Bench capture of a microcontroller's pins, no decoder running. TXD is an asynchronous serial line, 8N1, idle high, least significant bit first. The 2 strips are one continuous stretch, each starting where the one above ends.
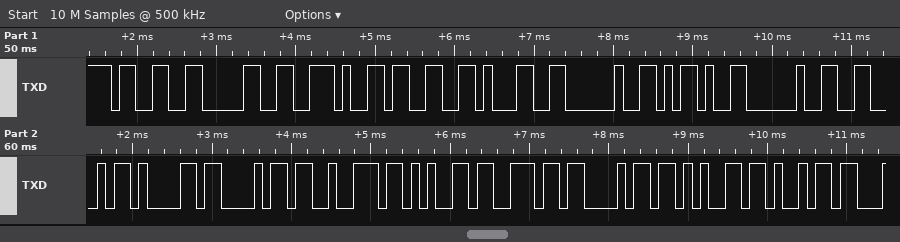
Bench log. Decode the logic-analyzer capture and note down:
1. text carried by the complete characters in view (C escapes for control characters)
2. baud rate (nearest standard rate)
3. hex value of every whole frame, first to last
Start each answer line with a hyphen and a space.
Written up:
- "30.31 - Fahrenhei"
- 9600 baud
- 33 30 2E 33 31 20 2D 20 46 61 68 72 65 6E 68 65 69
